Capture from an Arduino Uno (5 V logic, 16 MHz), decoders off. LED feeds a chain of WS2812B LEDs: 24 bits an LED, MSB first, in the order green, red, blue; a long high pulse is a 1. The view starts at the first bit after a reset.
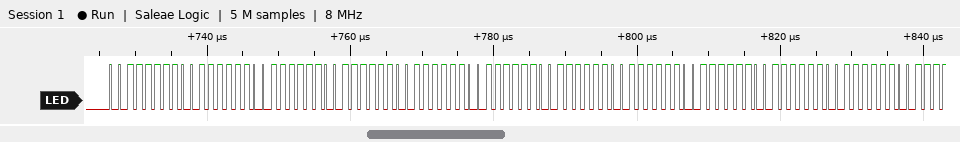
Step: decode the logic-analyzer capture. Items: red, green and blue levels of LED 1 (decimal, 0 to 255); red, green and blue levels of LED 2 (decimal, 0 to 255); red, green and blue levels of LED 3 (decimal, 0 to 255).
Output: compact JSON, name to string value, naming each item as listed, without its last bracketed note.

{"red, green and blue levels of LED 1": "63, 63, 63", "red, green and blue levels of LED 2": "63, 63, 63", "red, green and blue levels of LED 3": "63, 63, 63"}
